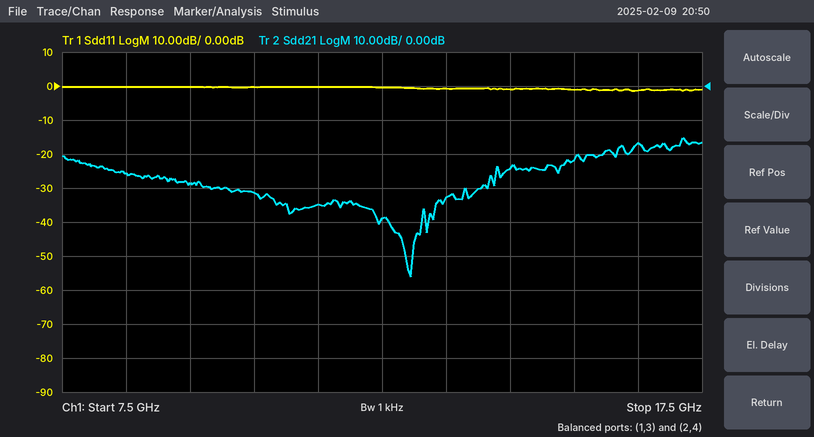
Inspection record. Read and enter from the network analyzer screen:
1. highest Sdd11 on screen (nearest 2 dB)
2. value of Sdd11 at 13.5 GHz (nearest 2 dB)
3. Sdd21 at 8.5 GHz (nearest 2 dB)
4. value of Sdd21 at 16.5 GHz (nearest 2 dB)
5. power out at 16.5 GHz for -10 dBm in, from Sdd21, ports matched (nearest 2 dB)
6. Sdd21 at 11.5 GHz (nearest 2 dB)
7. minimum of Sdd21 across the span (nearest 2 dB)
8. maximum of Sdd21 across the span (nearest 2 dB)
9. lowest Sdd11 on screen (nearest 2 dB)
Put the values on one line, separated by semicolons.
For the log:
0 dB; 0 dB; -26 dB; -16 dB; -26 dBm; -34 dB; -56 dB; -16 dB; -2 dB
